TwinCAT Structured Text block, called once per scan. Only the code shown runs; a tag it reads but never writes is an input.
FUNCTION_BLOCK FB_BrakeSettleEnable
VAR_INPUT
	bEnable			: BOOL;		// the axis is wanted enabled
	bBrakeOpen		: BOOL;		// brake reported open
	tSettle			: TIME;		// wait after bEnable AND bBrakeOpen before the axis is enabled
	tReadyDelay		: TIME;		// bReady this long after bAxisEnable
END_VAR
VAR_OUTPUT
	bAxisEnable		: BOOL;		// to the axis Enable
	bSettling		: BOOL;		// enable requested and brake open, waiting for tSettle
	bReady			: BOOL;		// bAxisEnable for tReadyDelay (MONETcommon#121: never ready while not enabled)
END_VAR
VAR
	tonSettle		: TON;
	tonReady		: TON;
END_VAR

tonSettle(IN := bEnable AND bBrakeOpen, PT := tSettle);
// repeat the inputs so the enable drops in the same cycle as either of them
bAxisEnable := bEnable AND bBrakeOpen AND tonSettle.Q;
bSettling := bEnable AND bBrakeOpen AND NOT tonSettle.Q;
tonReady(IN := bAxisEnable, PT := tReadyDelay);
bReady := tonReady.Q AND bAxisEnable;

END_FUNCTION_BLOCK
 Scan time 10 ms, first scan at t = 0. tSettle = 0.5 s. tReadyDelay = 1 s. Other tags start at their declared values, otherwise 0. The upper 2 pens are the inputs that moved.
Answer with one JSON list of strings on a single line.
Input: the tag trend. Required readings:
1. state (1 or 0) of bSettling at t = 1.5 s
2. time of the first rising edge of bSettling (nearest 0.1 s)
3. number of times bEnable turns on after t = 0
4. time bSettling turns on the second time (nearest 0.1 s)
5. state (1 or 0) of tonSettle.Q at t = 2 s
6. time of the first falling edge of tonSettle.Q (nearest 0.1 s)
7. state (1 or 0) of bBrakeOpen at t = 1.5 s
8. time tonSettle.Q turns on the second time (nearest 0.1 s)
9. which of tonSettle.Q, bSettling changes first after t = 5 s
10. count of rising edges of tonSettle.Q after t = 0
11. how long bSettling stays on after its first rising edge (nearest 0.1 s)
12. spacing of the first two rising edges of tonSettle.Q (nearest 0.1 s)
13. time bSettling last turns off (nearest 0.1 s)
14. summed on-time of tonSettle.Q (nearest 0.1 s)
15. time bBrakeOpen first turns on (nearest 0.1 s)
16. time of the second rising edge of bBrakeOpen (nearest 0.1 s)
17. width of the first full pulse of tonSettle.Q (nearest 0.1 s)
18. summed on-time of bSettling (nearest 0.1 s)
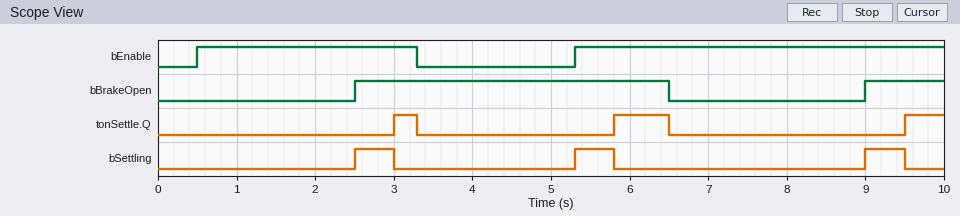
["0", "2.5 s", "2", "5.3 s", "0", "3.3 s", "0", "5.8 s", "bSettling", "3", "0.5 s", "2.8 s", "9.5 s", "1.5 s", "2.5 s", "9.0 s", "0.3 s", "1.5 s"]
